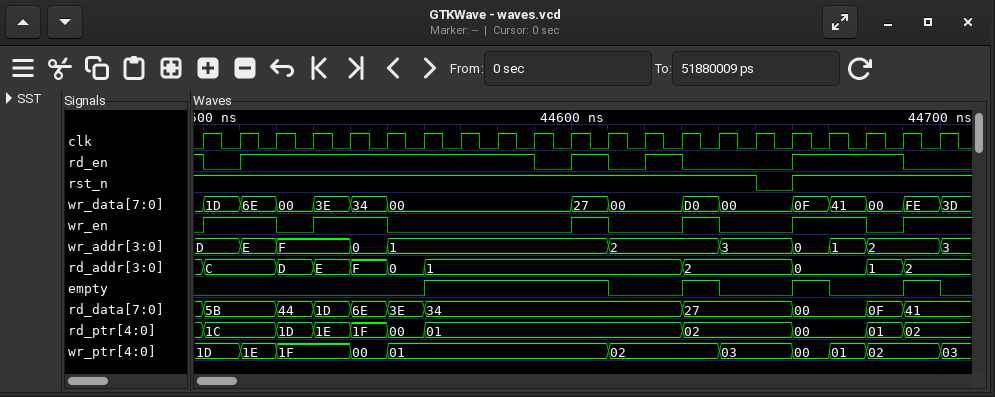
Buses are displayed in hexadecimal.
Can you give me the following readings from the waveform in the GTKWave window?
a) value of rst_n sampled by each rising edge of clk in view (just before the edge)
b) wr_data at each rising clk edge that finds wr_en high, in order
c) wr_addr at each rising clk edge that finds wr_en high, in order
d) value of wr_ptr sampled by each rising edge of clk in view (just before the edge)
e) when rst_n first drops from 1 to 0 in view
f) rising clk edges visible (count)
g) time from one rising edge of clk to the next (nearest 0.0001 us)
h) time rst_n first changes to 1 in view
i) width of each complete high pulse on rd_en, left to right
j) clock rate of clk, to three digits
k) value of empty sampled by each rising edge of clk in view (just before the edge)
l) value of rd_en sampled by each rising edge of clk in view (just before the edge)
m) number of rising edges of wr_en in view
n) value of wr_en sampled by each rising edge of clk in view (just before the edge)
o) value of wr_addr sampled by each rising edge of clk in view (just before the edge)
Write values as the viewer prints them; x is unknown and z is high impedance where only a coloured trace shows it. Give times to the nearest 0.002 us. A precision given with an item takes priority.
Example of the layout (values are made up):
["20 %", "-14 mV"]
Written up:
["1 1 1 1 1 1 1 1 1 1 1 1 1 1 1 1 0 1 1 1 1", "1D, 6E, 3E, 34, 27, D0, 0F, 41, FE", "D, E, F, 0, 1, 2, 0, 1, 2", "1D, 1D, 1E, 1F, 1F, 00, 01, 01, 01, 01, 01, 01, 02, 02, 02, 03, 03, 00, 01, 02, 02", "44.65 us", "21", "0.01 us", "44.66 us", "0.08 us, 0.01 us, 0.01 us, 0.03 us", "100 MHz", "0 0 0 0 0 0 0 1 1 1 1 1 0 0 1 0 0 1 0 0 1", "1 0 1 1 1 1 1 1 1 1 0 1 0 1 0 0 0 1 1 1 0", "6", "0 1 1 0 1 1 0 0 0 0 0 1 0 0 1 0 0 1 1 0 1", "D, D, E, F, F, 0, 1, 1, 1, 1, 1, 1, 2, 2, 2, 3, 3, 0, 1, 2, 2"]
